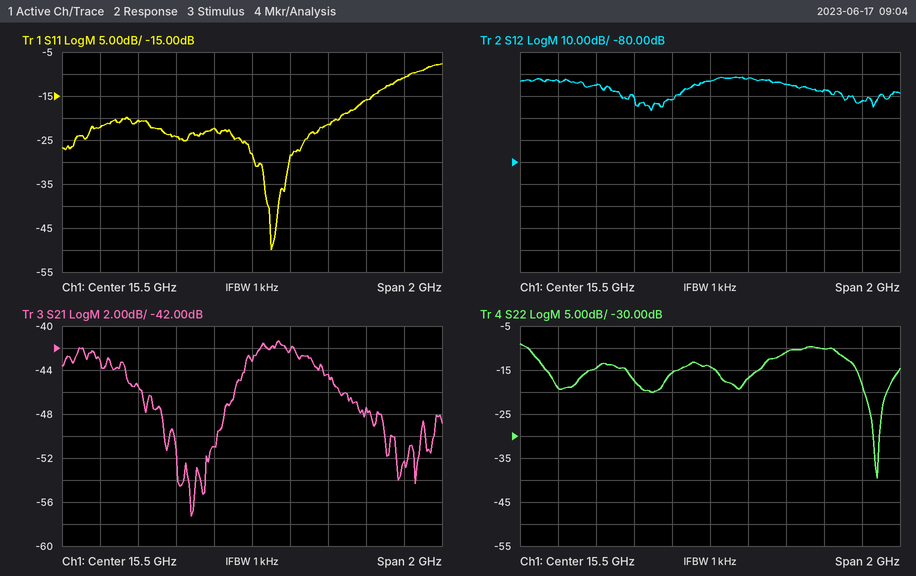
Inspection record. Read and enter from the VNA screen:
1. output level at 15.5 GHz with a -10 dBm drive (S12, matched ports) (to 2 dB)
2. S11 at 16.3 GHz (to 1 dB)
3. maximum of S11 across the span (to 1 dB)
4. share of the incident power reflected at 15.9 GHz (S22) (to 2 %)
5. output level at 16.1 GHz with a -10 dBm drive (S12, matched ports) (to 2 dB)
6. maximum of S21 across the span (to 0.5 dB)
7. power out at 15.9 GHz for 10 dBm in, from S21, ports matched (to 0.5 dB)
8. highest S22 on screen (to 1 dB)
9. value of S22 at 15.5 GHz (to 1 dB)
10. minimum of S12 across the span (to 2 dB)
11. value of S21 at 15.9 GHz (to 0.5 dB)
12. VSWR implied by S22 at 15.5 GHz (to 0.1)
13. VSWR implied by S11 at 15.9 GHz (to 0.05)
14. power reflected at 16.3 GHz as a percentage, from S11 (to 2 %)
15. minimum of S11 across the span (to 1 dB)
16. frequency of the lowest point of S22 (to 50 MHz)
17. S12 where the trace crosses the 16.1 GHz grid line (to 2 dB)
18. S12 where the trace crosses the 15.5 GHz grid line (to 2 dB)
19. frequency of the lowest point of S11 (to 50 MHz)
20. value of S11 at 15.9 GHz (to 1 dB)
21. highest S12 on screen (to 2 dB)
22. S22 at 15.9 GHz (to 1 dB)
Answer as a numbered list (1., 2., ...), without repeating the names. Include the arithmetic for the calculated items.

1. -10 dBm + (-44 dB) = -54 dBm
2. -11 dB
3. -8 dB
4. 10^(-11/10) ≈ 8 %
5. -10 dBm + (-48 dB) = -58 dBm
6. -41.5 dB
7. 10 dBm + (-44.5 dB) = -34.5 dBm
8. -9 dB
9. -14 dB
10. -56 dB
11. -44.5 dB
12. |Γ| = 10^(-14/20) = 0.1995; VSWR = (1 + 0.1995)/(1 − 0.1995) ≈ 1.5
13. |Γ| = 10^(-21/20) = 0.0891; VSWR = (1 + 0.0891)/(1 − 0.0891) ≈ 1.20
14. 10^(-11/10) ≈ 8 %
15. -50 dB
16. 16.40 GHz
17. -48 dB
18. -44 dB
19. 15.60 GHz
20. -21 dB
21. -42 dB
22. -11 dB
